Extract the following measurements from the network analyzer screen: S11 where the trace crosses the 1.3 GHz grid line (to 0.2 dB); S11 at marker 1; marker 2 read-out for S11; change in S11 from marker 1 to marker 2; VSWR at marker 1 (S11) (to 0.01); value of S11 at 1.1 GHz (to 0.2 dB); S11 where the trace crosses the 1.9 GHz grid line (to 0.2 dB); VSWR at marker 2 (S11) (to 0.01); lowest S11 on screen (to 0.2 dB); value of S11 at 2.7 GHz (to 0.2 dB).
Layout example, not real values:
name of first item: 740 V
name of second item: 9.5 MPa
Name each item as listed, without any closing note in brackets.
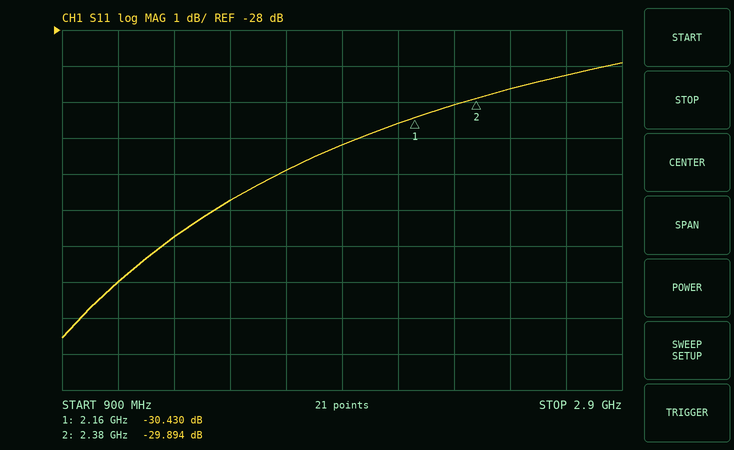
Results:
S11 where the trace crosses the 1.3 GHz grid line: -33.8 dB
S11 at marker 1: -30.430 dB
marker 2 read-out for S11: -29.894 dB
change in S11 from marker 1 to marker 2: 0.536 dB
VSWR at marker 1 (S11): 1.06
value of S11 at 1.1 GHz: -35.0 dB
S11 where the trace crosses the 1.9 GHz grid line: -31.2 dB
VSWR at marker 2 (S11): 1.07
lowest S11 on screen: -36.6 dB
value of S11 at 2.7 GHz: -29.2 dB
